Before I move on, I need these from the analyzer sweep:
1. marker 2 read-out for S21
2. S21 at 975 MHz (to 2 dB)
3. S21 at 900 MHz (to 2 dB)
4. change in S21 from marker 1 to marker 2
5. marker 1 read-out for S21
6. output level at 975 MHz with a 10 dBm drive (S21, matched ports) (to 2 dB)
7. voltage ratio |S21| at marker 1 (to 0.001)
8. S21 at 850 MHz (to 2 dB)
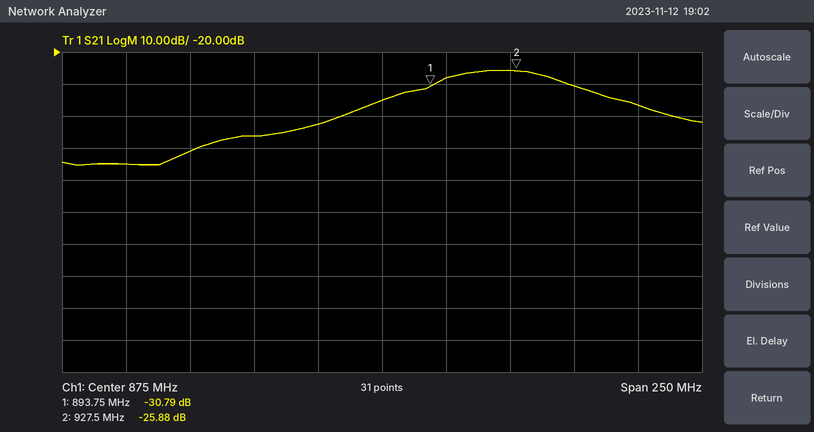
-25.88 dB
-36 dB
-28 dB
4.91 dB
-30.79 dB
-26 dBm
0.029
-42 dB
